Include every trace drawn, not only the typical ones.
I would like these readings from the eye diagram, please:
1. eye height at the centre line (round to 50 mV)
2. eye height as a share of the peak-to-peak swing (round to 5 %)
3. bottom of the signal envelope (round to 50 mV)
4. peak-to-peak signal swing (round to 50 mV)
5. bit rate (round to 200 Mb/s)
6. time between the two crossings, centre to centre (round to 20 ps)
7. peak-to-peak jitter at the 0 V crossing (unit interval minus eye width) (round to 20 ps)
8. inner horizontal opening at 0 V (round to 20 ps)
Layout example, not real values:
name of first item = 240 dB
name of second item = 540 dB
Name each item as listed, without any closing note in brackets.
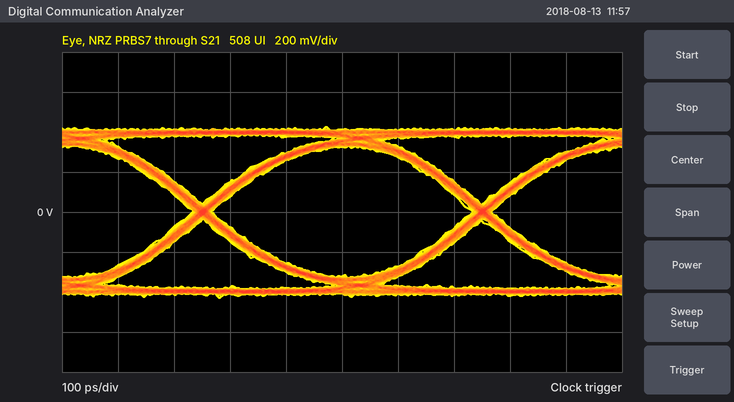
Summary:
eye height at the centre line = 650 mV
eye height as a share of the peak-to-peak swing = 75 %
bottom of the signal envelope = -450 mV
peak-to-peak signal swing = 850 mV
bit rate = 2.0 Gb/s
time between the two crossings, centre to centre = 500 ps
peak-to-peak jitter at the 0 V crossing (unit interval minus eye width) = 40 ps
inner horizontal opening at 0 V = 460 ps
